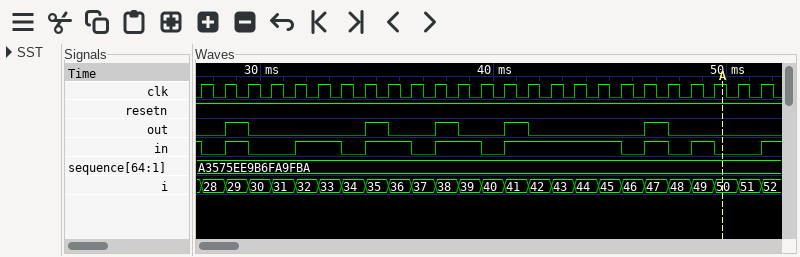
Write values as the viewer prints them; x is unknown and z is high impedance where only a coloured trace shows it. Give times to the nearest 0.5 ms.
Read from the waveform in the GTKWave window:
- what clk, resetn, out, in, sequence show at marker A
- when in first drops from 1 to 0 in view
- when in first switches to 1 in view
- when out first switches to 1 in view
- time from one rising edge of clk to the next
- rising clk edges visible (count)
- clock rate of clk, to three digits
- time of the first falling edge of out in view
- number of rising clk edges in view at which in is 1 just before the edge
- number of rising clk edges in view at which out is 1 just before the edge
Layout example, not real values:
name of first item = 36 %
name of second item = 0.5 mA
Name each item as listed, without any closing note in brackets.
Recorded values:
what clk, resetn, out, in, sequence show at marker A = clk=1, resetn=1, out=0, in=0, sequence=A3575EE9B6FA9FBA
when in first drops from 1 to 0 in view = 27.5 ms
when in first switches to 1 in view = 28.5 ms
when out first switches to 1 in view = 28.5 ms
time from one rising edge of clk to the next = 1 ms
rising clk edges visible = 25
clock rate of clk, to three digits = 1.00 kHz
time of the first falling edge of out in view = 29.5 ms
number of rising clk edges in view at which in is 1 just before the edge = 15
number of rising clk edges in view at which out is 1 just before the edge = 5
